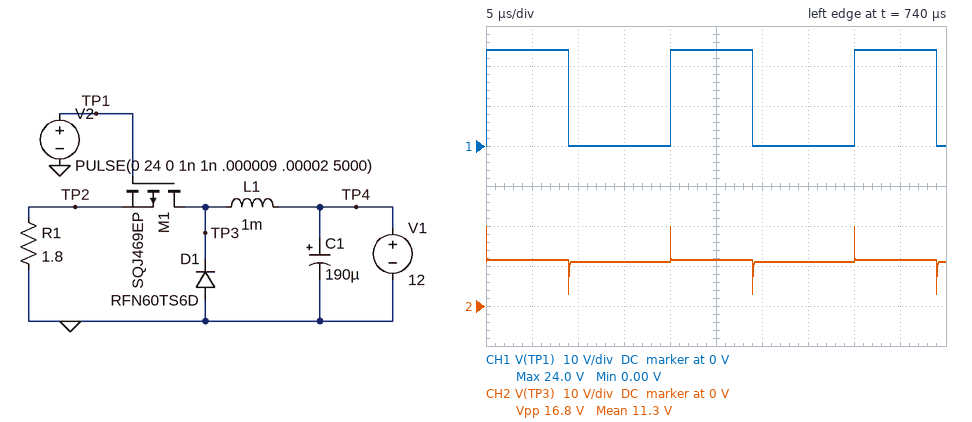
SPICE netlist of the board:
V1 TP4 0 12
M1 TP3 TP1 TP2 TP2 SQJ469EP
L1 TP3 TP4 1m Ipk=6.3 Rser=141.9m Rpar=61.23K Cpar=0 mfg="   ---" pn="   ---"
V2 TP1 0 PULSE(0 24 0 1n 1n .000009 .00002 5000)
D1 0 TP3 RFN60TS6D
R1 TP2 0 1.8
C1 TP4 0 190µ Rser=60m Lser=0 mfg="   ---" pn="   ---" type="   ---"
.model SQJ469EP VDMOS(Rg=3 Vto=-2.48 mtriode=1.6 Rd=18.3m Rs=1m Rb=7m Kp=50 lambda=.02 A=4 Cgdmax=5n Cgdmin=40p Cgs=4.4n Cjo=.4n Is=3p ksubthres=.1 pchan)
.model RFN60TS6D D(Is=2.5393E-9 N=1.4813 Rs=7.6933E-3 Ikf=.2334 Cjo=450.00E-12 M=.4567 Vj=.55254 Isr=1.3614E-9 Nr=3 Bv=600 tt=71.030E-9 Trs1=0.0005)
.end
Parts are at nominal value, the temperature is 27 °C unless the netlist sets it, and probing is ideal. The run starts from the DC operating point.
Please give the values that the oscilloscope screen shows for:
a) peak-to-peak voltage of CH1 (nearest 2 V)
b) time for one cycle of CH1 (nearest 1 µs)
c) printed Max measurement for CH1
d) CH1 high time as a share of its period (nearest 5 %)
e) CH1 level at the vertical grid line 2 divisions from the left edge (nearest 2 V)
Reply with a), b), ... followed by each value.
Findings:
a) 24 V
b) 20 µs
c) 24.0 V
d) 45 %
e) 0 V
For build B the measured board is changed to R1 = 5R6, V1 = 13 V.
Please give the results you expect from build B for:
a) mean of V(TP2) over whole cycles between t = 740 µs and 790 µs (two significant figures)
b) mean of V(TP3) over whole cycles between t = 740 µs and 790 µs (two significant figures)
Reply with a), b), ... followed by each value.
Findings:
a) 12 V
b) 13 V
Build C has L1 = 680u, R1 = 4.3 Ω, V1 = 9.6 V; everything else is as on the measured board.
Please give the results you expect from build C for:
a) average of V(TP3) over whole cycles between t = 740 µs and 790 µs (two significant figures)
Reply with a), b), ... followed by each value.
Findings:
a) 9.3 V
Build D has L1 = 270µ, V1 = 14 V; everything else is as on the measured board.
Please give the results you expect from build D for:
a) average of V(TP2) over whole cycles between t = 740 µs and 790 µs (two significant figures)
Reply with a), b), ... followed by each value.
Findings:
a) 13 V
